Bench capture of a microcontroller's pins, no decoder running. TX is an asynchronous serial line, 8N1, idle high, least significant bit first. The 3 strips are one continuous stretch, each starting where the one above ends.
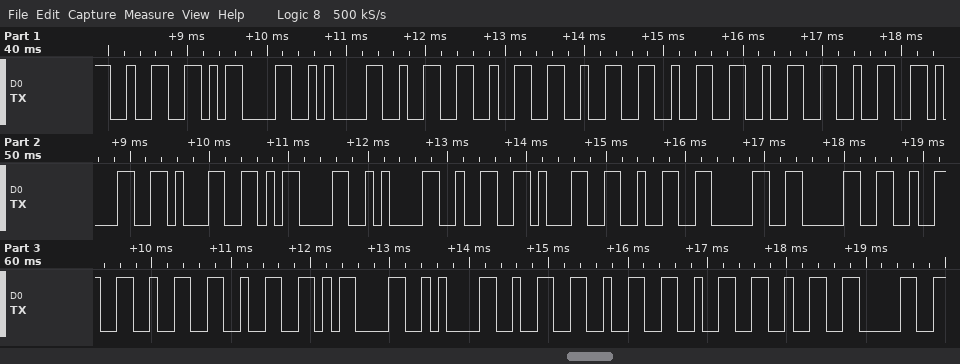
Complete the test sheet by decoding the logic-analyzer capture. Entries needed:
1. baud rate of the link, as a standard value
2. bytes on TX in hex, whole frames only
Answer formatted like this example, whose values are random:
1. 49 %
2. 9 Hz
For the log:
1. 9600 baud
2. 0x32 0x0D 0x0A 0x32 0x32 0x32 0x32 0x32 0x32 0x31 0x31 0x0D 0x0A 0x32 0x31 0x32 0x30 0x30 0x32 0x32 0x32 0x0D 0x0A 0x32 0x32 0x32 0x32 0x30
